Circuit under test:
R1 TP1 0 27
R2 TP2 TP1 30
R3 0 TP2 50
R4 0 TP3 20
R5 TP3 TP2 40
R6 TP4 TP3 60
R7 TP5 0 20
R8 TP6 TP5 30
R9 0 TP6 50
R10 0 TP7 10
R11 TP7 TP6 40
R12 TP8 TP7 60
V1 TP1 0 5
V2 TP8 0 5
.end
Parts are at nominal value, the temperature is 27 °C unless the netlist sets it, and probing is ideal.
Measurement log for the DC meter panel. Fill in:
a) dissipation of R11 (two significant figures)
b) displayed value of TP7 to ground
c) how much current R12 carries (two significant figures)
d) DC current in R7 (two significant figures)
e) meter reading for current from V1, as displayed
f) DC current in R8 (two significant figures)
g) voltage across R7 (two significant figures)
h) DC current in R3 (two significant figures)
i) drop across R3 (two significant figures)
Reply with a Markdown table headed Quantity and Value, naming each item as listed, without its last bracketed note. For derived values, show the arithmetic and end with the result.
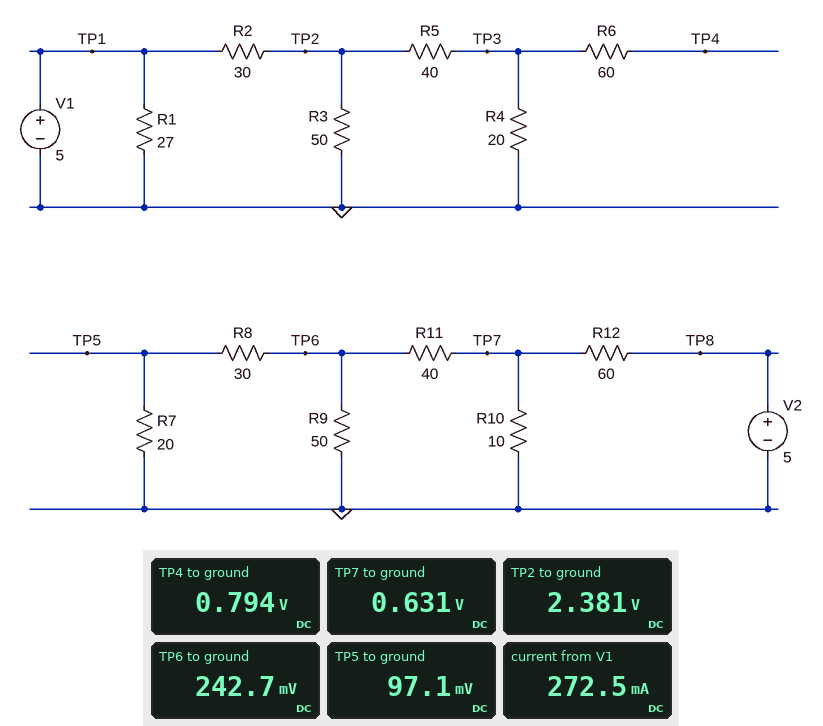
| Quantity | Value |
|---|---|
| dissipation of R11 | (631 mV - 242.7 mV)^2 / 40 Ω = 3.8 mW |
| displayed value of TP7 to ground | 0.631 V |
| how much current R12 carries | (5 V - 631 mV) / 60 Ω = 73 mA |
| DC current in R7 | (97.1 mV) / 20 Ω = 4.9 mA |
| meter reading for current from V1, as displayed | 272.5 mA |
| DC current in R8 | (242.7 mV - 97.1 mV) / 30 Ω = 4.9 mA |
| voltage across R7 | 97.1 mV = 97 mV |
| DC current in R3 | (2.381 V) / 50 Ω = 48 mA |
| drop across R3 | 2.381 V = 2.4 V |
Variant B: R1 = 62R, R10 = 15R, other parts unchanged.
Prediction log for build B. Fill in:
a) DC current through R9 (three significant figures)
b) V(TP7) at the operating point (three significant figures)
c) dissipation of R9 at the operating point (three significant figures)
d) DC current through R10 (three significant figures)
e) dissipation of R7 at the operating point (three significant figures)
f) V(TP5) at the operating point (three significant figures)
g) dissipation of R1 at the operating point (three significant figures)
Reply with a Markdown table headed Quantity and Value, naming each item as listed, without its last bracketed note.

| Quantity | Value |
|---|---|
| DC current through R9 | 6.49 mA |
| V(TP7) at the operating point | 844 mV |
| dissipation of R9 at the operating point | 2.11 mW |
| DC current through R10 | 56.3 mA |
| dissipation of R7 at the operating point | 843 µW |
| V(TP5) at the operating point | 130 mV |
| dissipation of R1 at the operating point | 403 mW |
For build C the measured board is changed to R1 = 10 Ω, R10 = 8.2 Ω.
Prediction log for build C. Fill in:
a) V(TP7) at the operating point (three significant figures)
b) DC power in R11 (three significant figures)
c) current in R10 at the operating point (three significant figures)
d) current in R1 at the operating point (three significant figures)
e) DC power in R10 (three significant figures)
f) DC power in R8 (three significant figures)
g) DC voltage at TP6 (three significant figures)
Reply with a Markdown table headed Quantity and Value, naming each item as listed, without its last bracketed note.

| Quantity | Value |
|---|---|
| V(TP7) at the operating point | 541 mV |
| DC power in R11 | 2.77 mW |
| current in R10 at the operating point | 66.0 mA |
| current in R1 at the operating point | 500 mA |
| DC power in R10 | 35.7 mW |
| DC power in R8 | 520 µW |
| DC voltage at TP6 | 208 mV |
